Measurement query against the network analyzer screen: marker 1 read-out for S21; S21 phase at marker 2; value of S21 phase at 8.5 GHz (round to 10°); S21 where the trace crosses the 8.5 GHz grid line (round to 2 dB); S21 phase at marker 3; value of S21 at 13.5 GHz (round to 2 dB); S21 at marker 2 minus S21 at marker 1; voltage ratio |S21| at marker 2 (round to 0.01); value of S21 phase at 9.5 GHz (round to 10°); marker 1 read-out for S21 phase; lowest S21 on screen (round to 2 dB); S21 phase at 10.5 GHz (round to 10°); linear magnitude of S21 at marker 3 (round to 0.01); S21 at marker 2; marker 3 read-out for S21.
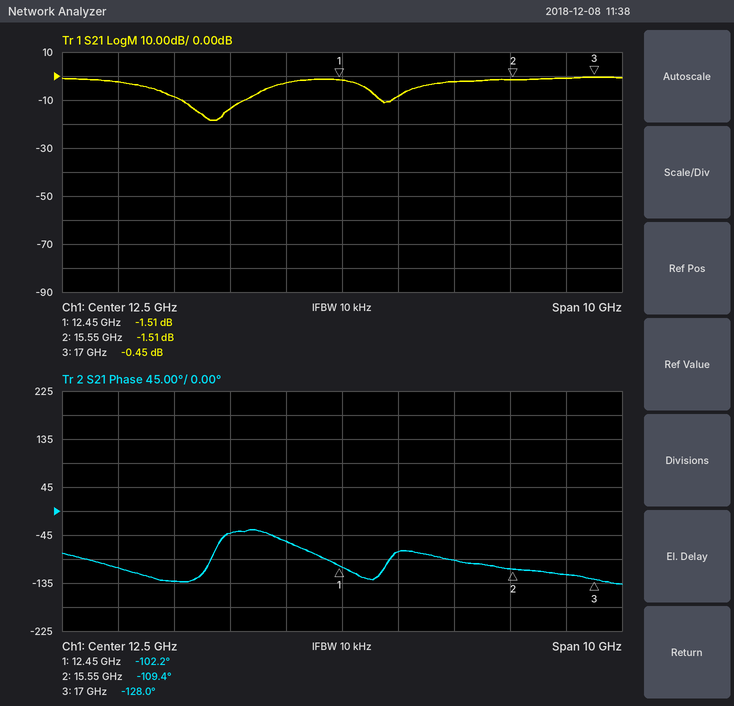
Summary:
-1.51 dB
-109.4°
-110°
-2 dB
-128.0°
-8 dB
0.00 dB
0.84
-130°
-102.2°
-18 dB
-40°
0.95
-1.51 dB
-0.45 dB
